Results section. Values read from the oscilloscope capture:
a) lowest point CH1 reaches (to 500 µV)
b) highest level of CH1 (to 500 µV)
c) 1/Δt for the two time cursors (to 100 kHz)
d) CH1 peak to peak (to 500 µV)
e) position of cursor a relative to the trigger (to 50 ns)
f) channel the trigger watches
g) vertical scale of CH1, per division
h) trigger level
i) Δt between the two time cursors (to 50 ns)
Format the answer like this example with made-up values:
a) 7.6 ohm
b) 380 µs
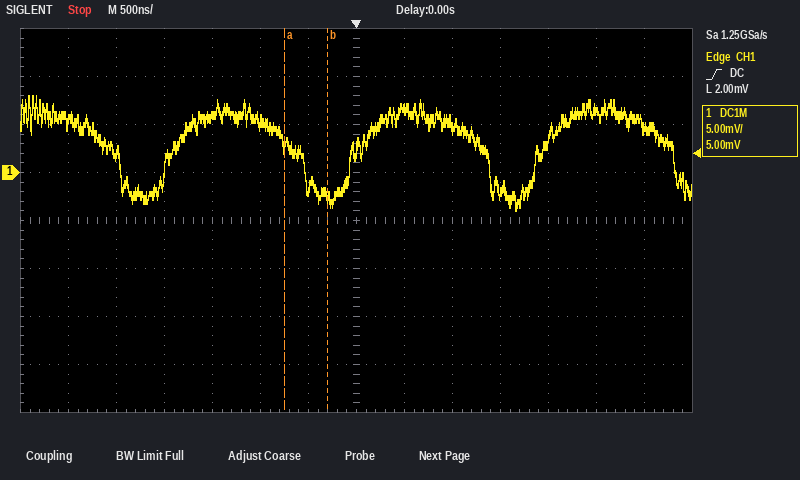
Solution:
a) -4.0 mV
b) 8.0 mV
c) 2.2 MHz
d) 12.0 mV
e) -750 ns
f) CH1
g) 5 mV
h) 2.00 mV
i) 450 ns
